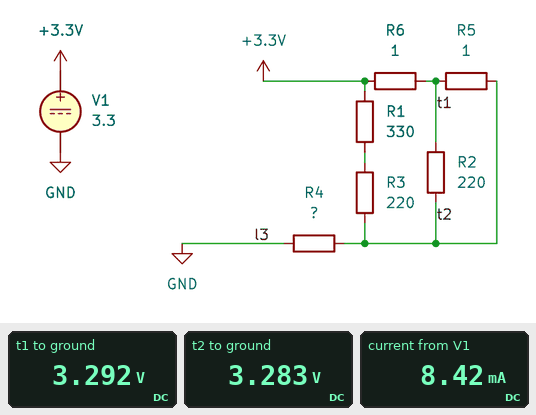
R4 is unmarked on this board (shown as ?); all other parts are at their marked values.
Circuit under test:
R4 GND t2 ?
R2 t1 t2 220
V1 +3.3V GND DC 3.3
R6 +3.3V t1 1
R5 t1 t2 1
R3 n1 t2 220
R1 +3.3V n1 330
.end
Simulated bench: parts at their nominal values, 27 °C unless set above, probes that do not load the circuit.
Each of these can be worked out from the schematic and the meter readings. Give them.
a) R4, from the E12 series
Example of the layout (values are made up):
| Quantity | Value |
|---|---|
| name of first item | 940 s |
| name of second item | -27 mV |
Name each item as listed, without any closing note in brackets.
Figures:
| Quantity | Value |
|---|---|
| R4, from the E12 series | 390 Ω |
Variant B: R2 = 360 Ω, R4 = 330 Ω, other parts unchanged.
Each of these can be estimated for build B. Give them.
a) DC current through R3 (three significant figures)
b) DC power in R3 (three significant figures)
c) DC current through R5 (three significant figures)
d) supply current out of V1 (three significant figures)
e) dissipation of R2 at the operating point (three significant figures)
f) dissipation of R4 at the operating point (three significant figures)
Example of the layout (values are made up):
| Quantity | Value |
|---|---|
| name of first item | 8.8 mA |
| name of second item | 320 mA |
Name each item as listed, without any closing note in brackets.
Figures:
| Quantity | Value |
|---|---|
| DC current through R3 | 36.0 µA |
| DC power in R3 | 285 nW |
| DC current through R5 | 9.88 mA |
| supply current out of V1 | 9.94 mA |
| dissipation of R2 at the operating point | 271 nW |
| dissipation of R4 at the operating point | 32.6 mW |
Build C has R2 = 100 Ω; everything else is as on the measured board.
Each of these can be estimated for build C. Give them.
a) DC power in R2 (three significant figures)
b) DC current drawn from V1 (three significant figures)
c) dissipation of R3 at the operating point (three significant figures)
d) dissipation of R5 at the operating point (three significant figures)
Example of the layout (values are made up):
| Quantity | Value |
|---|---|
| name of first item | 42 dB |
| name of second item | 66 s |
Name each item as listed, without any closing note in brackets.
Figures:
| Quantity | Value |
|---|---|
| DC power in R2 | 690 nW |
| DC current drawn from V1 | 8.42 mA |
| dissipation of R3 at the operating point | 203 nW |
| dissipation of R5 at the operating point | 69.0 µW |
